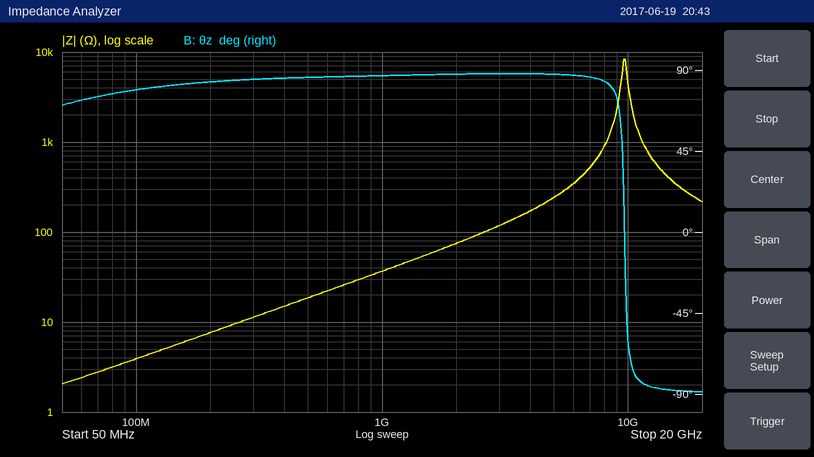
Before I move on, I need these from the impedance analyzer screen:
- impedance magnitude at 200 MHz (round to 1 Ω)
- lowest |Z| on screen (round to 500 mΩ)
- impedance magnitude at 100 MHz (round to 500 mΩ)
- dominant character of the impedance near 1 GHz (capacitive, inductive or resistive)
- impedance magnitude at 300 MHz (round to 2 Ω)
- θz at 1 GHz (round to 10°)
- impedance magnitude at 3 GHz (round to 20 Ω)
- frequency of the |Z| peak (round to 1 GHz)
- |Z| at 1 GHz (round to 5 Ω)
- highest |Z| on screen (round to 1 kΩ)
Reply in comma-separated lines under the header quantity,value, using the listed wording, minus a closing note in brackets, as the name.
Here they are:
quantity,value
impedance magnitude at 200 MHz,8 Ω
lowest |Z| on screen,2.0 Ω
impedance magnitude at 100 MHz,4.0 Ω
dominant character of the impedance near 1 GHz,inductive
impedance magnitude at 300 MHz,12 Ω
θz at 1 GHz,90°
impedance magnitude at 3 GHz,120 Ω
frequency of the |Z| peak,10 GHz
|Z| at 1 GHz,35 Ω
highest |Z| on screen,8 kΩ
